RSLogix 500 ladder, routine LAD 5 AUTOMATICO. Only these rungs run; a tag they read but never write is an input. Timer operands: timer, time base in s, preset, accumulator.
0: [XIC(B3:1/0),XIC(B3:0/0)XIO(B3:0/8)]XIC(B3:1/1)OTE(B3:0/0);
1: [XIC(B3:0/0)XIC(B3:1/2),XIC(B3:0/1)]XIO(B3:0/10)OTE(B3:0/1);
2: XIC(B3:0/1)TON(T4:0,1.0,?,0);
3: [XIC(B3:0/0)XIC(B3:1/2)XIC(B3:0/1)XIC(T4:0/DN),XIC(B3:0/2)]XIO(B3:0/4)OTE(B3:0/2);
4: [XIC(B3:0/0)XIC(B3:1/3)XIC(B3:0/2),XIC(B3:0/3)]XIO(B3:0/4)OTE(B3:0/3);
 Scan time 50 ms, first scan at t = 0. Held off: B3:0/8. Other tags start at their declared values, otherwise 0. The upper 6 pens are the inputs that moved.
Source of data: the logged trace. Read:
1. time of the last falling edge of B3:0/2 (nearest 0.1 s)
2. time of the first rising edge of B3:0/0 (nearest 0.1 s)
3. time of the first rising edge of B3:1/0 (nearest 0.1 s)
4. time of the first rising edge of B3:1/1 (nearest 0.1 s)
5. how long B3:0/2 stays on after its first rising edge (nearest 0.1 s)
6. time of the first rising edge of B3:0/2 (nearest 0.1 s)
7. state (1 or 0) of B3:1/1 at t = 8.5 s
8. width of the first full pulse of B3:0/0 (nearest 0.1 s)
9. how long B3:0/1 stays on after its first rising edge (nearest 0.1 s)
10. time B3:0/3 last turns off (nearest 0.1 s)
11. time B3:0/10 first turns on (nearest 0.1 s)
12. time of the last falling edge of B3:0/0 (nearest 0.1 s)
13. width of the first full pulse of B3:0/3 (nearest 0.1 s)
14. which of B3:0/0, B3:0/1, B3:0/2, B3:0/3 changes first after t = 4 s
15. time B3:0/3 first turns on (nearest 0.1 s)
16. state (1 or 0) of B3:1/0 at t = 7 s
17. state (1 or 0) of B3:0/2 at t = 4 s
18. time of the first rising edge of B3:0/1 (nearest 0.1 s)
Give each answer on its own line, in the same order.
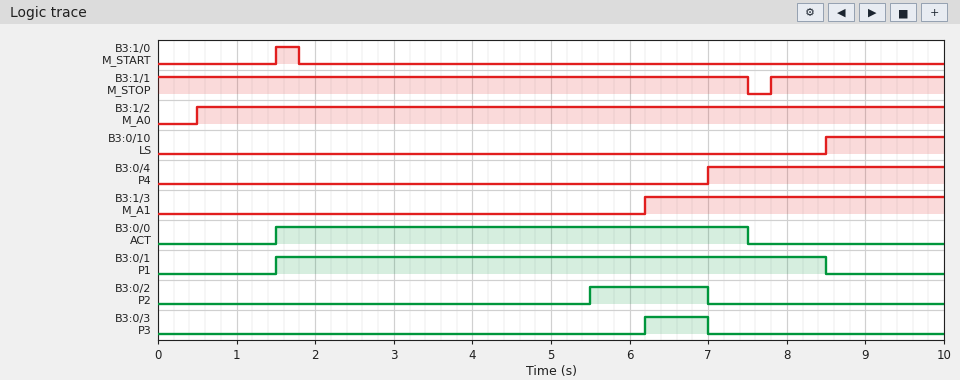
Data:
7.0 s
1.5 s
1.5 s
7.8 s
1.5 s
5.5 s
1
6.0 s
7.0 s
7.0 s
8.5 s
7.5 s
0.8 s
B3:0/2
6.2 s
0
0
1.5 s
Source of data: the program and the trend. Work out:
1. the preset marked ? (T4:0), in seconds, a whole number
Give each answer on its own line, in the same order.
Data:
4 s
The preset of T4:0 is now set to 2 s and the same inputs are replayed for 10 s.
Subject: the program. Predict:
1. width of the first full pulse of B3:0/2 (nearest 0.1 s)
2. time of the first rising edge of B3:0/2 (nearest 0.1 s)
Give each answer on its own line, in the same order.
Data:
3.5 s
3.5 s
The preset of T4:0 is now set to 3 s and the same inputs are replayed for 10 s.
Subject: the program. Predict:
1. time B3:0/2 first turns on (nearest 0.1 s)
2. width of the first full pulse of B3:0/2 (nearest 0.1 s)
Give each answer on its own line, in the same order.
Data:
4.5 s
2.5 s
